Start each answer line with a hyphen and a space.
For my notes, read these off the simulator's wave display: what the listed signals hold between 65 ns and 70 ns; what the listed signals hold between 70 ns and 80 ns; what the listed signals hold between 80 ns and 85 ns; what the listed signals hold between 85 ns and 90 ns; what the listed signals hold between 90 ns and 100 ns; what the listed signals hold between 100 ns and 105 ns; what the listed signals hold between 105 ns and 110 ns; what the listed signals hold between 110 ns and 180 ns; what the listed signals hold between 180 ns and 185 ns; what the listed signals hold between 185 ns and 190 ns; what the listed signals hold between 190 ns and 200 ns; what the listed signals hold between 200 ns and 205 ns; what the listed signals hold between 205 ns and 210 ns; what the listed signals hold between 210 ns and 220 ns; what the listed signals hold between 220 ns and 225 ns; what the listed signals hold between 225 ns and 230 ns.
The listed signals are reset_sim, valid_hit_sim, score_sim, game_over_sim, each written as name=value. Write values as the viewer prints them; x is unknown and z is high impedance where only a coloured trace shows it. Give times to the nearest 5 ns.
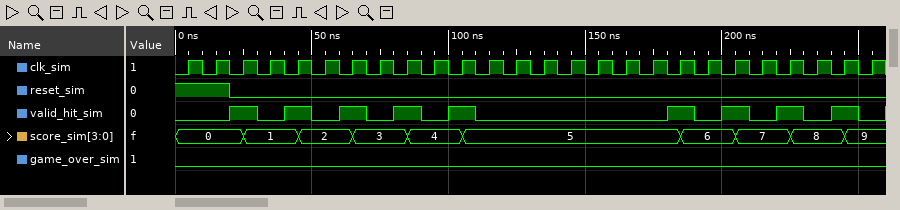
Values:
- reset_sim=0, valid_hit_sim=1, score_sim=3, game_over_sim=0
- reset_sim=0, valid_hit_sim=0, score_sim=3, game_over_sim=0
- reset_sim=0, valid_hit_sim=1, score_sim=3, game_over_sim=0
- reset_sim=0, valid_hit_sim=1, score_sim=4, game_over_sim=0
- reset_sim=0, valid_hit_sim=0, score_sim=4, game_over_sim=0
- reset_sim=0, valid_hit_sim=1, score_sim=4, game_over_sim=0
- reset_sim=0, valid_hit_sim=1, score_sim=5, game_over_sim=0
- reset_sim=0, valid_hit_sim=0, score_sim=5, game_over_sim=0
- reset_sim=0, valid_hit_sim=1, score_sim=5, game_over_sim=0
- reset_sim=0, valid_hit_sim=1, score_sim=6, game_over_sim=0
- reset_sim=0, valid_hit_sim=0, score_sim=6, game_over_sim=0
- reset_sim=0, valid_hit_sim=1, score_sim=6, game_over_sim=0
- reset_sim=0, valid_hit_sim=1, score_sim=7, game_over_sim=0
- reset_sim=0, valid_hit_sim=0, score_sim=7, game_over_sim=0
- reset_sim=0, valid_hit_sim=1, score_sim=7, game_over_sim=0
- reset_sim=0, valid_hit_sim=1, score_sim=8, game_over_sim=0
